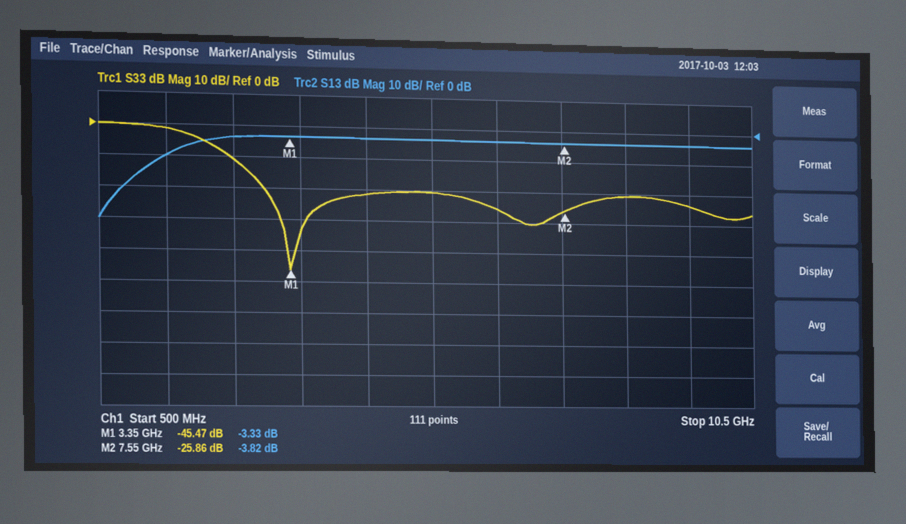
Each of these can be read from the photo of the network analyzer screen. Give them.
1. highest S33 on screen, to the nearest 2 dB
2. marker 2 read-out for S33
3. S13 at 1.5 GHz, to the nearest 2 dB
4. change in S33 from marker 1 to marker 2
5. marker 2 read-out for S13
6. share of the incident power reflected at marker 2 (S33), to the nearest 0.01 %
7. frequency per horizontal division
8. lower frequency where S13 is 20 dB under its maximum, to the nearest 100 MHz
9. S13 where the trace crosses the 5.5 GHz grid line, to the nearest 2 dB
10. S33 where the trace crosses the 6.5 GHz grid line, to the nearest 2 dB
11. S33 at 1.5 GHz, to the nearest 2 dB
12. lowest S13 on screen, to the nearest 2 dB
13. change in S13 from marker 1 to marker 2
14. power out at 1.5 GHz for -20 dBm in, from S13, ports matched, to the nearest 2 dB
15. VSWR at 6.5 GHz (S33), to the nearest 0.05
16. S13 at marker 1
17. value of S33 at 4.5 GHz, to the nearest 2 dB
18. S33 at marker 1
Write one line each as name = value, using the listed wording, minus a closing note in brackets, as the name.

highest S33 on screen, to the nearest 2 dB = 0 dB
marker 2 read-out for S33 = -25.86 dB
S13 at 1.5 GHz, to the nearest 2 dB = -10 dB
change in S33 from marker 1 to marker 2 = 19.61 dB
marker 2 read-out for S13 = -3.82 dB
share of the incident power reflected at marker 2 (S33), to the nearest 0.01 % = 0.26 %
frequency per horizontal division = 1 GHz
lower frequency where S13 is 20 dB under its maximum, to the nearest 100 MHz = 700 MHz
S13 where the trace crosses the 5.5 GHz grid line, to the nearest 2 dB = -4 dB
S33 where the trace crosses the 6.5 GHz grid line, to the nearest 2 dB = -26 dB
S33 at 1.5 GHz, to the nearest 2 dB = -2 dB
lowest S13 on screen, to the nearest 2 dB = -30 dB
change in S13 from marker 1 to marker 2 = -0.49 dB
power out at 1.5 GHz for -20 dBm in, from S13, ports matched, to the nearest 2 dB = -30 dBm
VSWR at 6.5 GHz (S33), to the nearest 0.05 = 1.10
S13 at marker 1 = -3.33 dB
value of S33 at 4.5 GHz, to the nearest 2 dB = -22 dB
S33 at marker 1 = -45.47 dB
